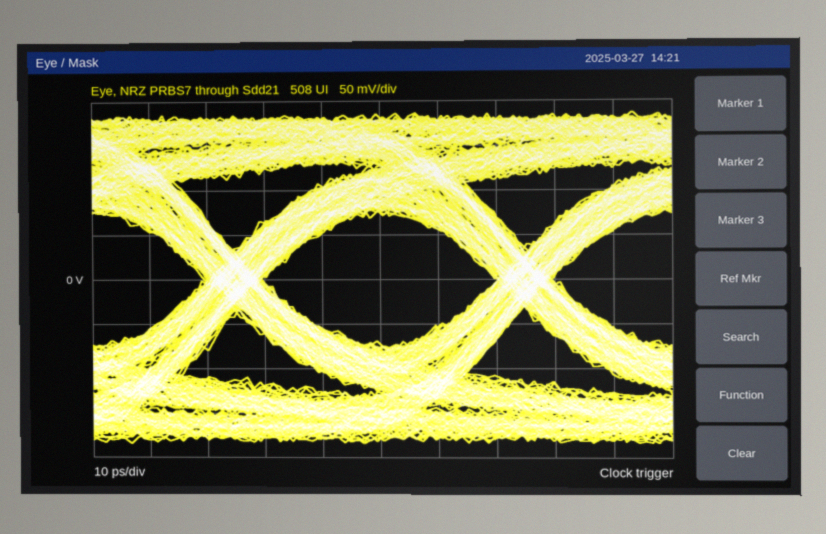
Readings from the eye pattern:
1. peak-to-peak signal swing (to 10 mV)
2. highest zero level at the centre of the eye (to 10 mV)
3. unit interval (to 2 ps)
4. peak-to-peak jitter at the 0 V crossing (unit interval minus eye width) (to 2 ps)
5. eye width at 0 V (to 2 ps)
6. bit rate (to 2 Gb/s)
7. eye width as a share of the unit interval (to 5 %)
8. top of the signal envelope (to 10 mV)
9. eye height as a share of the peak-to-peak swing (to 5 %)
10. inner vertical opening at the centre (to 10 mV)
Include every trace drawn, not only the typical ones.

370 mV
-70 mV
50 ps
10 ps
40 ps
20 Gb/s
80 %
190 mV
40 %
150 mV
